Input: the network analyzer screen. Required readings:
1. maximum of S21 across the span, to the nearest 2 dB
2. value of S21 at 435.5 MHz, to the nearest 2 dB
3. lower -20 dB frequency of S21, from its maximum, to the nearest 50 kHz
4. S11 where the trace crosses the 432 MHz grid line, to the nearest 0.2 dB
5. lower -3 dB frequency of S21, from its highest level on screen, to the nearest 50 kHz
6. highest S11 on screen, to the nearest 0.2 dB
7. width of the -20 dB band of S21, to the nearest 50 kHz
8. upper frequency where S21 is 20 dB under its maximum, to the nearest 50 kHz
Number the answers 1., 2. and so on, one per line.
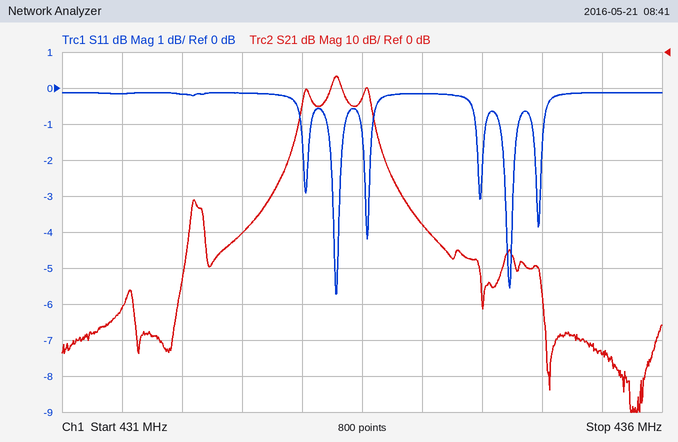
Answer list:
1. -6 dB
2. -84 dB
3. 432.90 MHz
4. -0.2 dB
5. 433.25 MHz
6. -0.2 dB
7. 750 kHz
8. 433.65 MHz
